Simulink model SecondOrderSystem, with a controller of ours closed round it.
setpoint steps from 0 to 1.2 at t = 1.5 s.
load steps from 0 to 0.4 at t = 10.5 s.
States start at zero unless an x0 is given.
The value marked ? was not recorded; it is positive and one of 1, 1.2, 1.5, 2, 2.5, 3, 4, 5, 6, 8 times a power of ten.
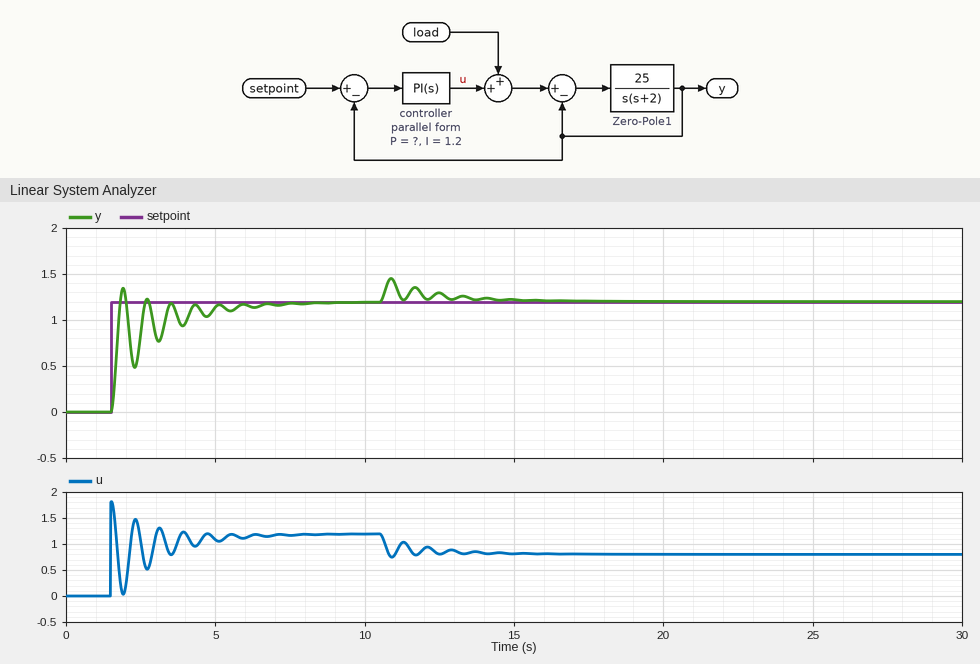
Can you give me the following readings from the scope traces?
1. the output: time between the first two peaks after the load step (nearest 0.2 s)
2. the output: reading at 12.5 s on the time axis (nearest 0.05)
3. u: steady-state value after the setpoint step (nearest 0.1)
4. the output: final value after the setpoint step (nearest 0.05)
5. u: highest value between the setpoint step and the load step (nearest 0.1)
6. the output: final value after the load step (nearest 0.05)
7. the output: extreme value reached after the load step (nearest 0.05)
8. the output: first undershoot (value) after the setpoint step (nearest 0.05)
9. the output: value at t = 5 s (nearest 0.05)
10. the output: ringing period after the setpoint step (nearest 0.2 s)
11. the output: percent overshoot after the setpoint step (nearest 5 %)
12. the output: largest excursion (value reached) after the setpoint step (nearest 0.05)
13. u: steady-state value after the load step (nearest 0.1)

0.8 s
1.30
1.2
1.20
1.8
1.20
1.45
0.50
1.15
0.8 s
10 %
1.35
0.8
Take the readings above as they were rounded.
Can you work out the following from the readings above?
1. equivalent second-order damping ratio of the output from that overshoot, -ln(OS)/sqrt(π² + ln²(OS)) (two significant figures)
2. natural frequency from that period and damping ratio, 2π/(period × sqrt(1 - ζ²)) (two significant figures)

0.59
9.7 rad/s
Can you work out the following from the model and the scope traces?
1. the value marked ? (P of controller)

1.5
